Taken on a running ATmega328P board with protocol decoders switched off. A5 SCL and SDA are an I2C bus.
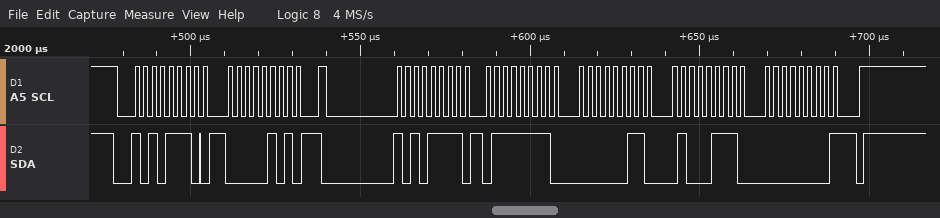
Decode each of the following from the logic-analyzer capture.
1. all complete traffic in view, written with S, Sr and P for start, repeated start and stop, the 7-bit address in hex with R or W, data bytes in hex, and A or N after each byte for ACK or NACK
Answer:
S 57W A 05 A Sr 57R A 7F A 03 A 47 A 00 N P
